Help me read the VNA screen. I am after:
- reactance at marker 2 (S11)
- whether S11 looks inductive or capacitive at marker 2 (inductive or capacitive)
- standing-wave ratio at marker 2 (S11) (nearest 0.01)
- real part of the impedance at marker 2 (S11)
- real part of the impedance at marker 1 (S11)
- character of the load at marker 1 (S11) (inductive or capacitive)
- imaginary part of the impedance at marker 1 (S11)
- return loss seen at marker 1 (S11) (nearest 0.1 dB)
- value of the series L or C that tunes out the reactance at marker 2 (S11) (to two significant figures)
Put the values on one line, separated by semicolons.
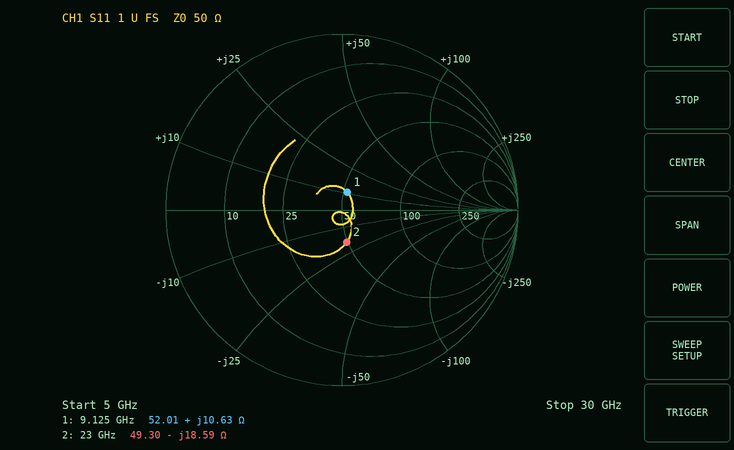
-18.59 Ω; capacitive; 1.45; 49.30 Ω; 52.01 Ω; inductive; +10.63 Ω; 19.5 dB; 130 pH
